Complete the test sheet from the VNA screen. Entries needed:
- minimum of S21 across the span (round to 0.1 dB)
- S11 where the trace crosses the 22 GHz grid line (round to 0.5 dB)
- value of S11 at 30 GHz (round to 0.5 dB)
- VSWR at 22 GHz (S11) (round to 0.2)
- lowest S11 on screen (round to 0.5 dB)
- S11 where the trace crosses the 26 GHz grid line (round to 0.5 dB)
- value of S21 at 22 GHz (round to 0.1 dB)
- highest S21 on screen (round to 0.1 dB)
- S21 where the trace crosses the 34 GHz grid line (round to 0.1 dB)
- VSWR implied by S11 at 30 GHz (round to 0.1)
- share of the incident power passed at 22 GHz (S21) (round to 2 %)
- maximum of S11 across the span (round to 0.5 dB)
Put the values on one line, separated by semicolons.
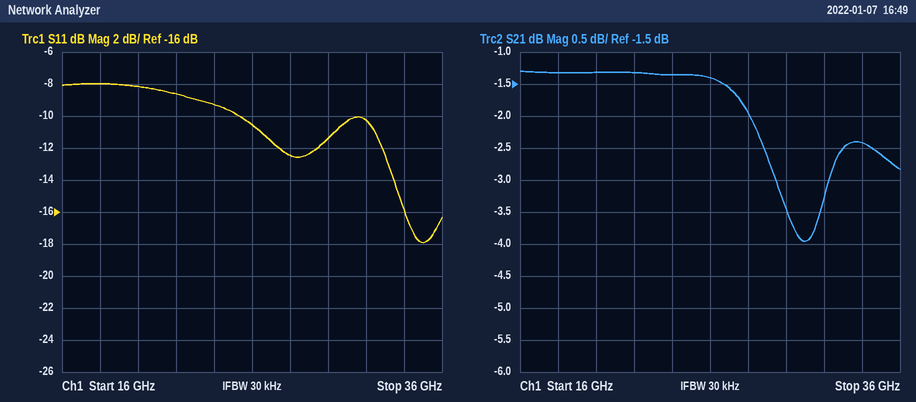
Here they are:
-4.0 dB; -8.5 dB; -11.5 dB; 2.2; -18.0 dB; -10.5 dB; -1.3 dB; -1.3 dB; -2.4 dB; 1.7; 74 %; -8.0 dB
